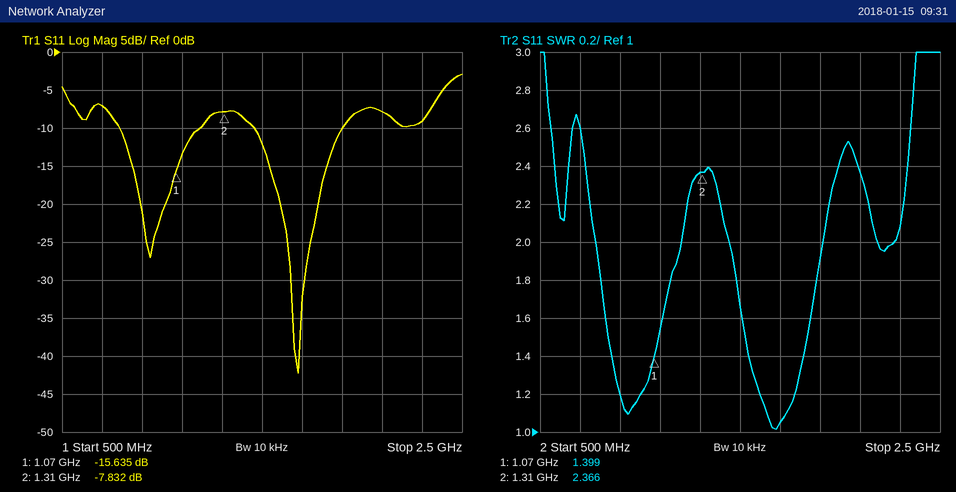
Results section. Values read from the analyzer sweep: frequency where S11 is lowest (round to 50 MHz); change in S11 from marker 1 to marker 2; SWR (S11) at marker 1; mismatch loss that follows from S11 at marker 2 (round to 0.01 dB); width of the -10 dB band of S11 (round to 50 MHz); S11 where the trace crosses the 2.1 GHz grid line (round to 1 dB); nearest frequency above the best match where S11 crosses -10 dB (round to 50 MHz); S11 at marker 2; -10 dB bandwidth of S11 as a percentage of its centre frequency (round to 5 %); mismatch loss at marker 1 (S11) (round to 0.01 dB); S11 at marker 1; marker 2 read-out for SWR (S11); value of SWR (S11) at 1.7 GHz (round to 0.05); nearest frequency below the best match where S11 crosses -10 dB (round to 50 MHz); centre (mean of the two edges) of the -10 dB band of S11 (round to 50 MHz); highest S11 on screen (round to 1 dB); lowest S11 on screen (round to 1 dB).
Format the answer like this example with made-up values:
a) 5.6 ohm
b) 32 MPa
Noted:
a) 1.70 GHz
b) 7.803 dB
c) 1.399
d) 0.78 dB
e) 450 MHz
f) -8 dB
g) 1.90 GHz
h) -7.832 dB
i) 25 %
j) 0.12 dB
k) -15.635 dB
l) 2.366
m) 1.05
n) 1.45 GHz
o) 1.70 GHz
p) -3 dB
q) -42 dB
